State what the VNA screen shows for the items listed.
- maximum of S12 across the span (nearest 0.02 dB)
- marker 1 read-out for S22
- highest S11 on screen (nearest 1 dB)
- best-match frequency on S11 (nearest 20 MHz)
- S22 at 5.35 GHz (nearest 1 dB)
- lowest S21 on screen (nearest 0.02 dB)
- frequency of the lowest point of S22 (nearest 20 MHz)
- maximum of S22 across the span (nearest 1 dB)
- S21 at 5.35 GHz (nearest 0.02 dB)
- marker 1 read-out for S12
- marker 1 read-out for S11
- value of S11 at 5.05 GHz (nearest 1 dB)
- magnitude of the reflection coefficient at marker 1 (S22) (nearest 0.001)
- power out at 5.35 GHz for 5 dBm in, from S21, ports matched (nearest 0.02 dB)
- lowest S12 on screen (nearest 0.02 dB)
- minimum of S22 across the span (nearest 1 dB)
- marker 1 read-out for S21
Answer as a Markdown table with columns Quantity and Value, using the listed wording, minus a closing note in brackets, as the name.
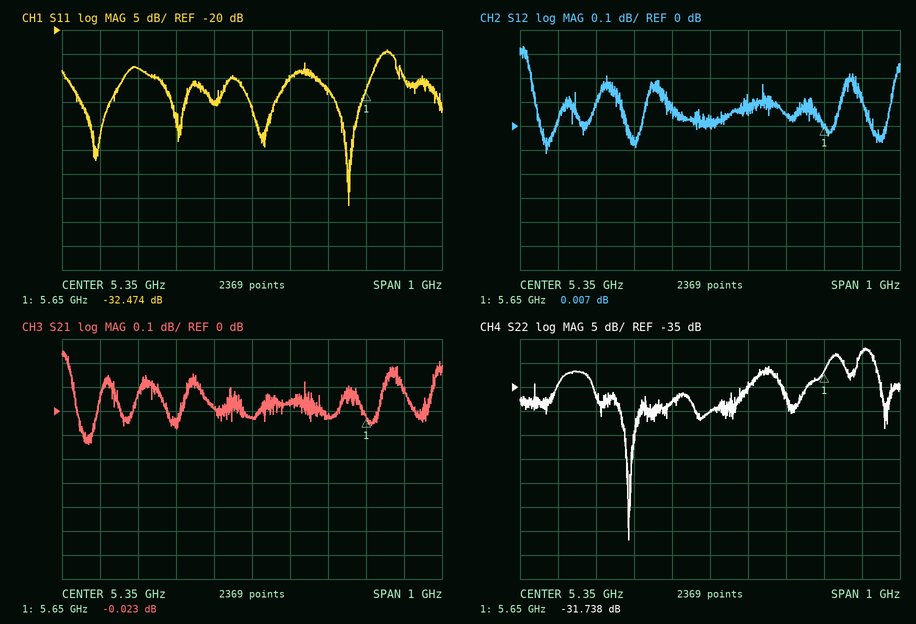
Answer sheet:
| Quantity | Value |
|---|---|
| maximum of S12 across the span | 0.34 dB |
| marker 1 read-out for S22 | -31.738 dB |
| highest S11 on screen | -24 dB |
| best-match frequency on S11 | 5.60 GHz |
| S22 at 5.35 GHz | -40 dB |
| lowest S21 on screen | -0.14 dB |
| frequency of the lowest point of S22 | 5.14 GHz |
| maximum of S22 across the span | -27 dB |
| S21 at 5.35 GHz | -0.02 dB |
| marker 1 read-out for S12 | 0.007 dB |
| marker 1 read-out for S11 | -32.474 dB |
| value of S11 at 5.05 GHz | -28 dB |
| magnitude of the reflection coefficient at marker 1 (S22) | 0.026 |
| power out at 5.35 GHz for 5 dBm in, from S21, ports matched | 4.98 dBm |
| lowest S12 on screen | -0.12 dB |
| minimum of S22 across the span | -67 dB |
| marker 1 read-out for S21 | -0.023 dB |
